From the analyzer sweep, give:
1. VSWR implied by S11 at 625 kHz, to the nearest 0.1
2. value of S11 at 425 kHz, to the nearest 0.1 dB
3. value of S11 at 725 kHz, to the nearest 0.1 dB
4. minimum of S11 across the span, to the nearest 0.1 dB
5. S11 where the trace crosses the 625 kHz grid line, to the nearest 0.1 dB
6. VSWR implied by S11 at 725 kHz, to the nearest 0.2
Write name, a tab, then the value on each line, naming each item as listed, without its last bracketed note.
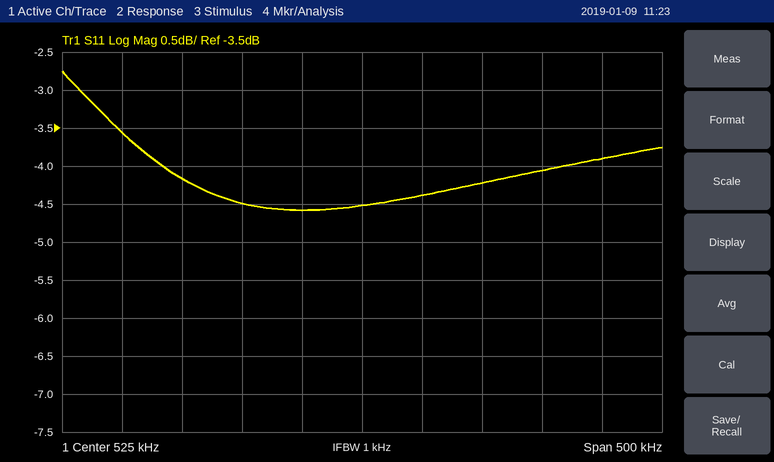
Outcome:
VSWR implied by S11 at 625 kHz, to the nearest 0.1	4.2
value of S11 at 425 kHz, to the nearest 0.1 dB	-4.5 dB
value of S11 at 725 kHz, to the nearest 0.1 dB	-3.9 dB
minimum of S11 across the span, to the nearest 0.1 dB	-4.6 dB
S11 where the trace crosses the 625 kHz grid line, to the nearest 0.1 dB	-4.2 dB
VSWR implied by S11 at 725 kHz, to the nearest 0.2	4.6
